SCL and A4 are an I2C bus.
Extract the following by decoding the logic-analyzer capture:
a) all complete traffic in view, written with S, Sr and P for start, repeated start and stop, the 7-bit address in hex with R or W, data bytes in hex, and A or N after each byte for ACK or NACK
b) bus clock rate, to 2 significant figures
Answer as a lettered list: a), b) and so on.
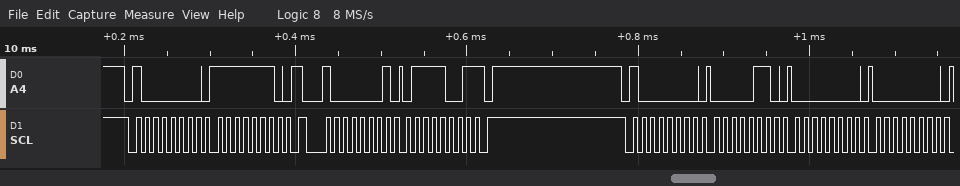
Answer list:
a) S 40W A FE A Sr 40R A 79 N P S 40W A 06 A 00 A 00 A
b) 100 kHz
